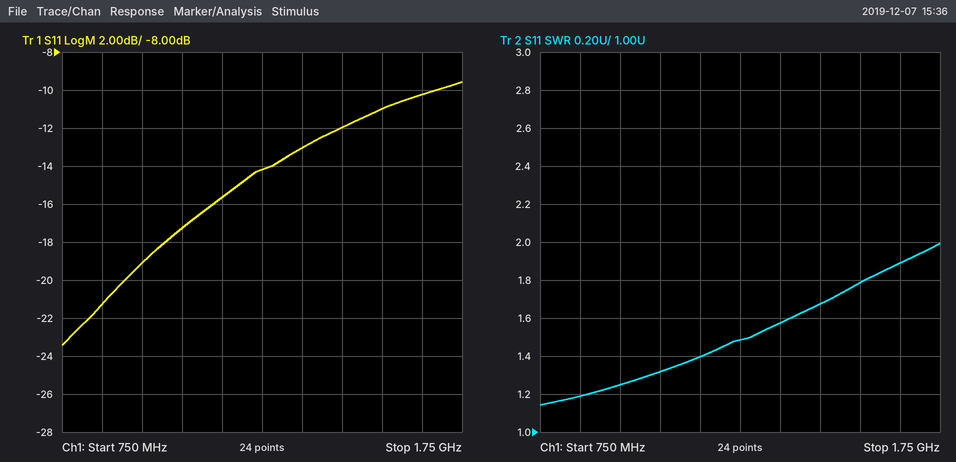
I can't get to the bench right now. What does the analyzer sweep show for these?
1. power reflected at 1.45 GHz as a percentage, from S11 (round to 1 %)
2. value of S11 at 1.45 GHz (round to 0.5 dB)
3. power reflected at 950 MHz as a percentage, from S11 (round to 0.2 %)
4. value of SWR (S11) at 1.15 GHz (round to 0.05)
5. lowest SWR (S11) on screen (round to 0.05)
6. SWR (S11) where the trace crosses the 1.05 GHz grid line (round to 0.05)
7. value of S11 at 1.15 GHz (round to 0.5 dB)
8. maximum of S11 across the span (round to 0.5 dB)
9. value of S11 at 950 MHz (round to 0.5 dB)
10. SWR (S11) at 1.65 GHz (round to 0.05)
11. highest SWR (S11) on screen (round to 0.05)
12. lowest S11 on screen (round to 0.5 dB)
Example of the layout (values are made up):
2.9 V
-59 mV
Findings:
6 %
-12.0 dB
1.2 %
1.40
1.15
1.30
-15.5 dB
-9.5 dB
-19.0 dB
1.90
2.00
-23.5 dB
